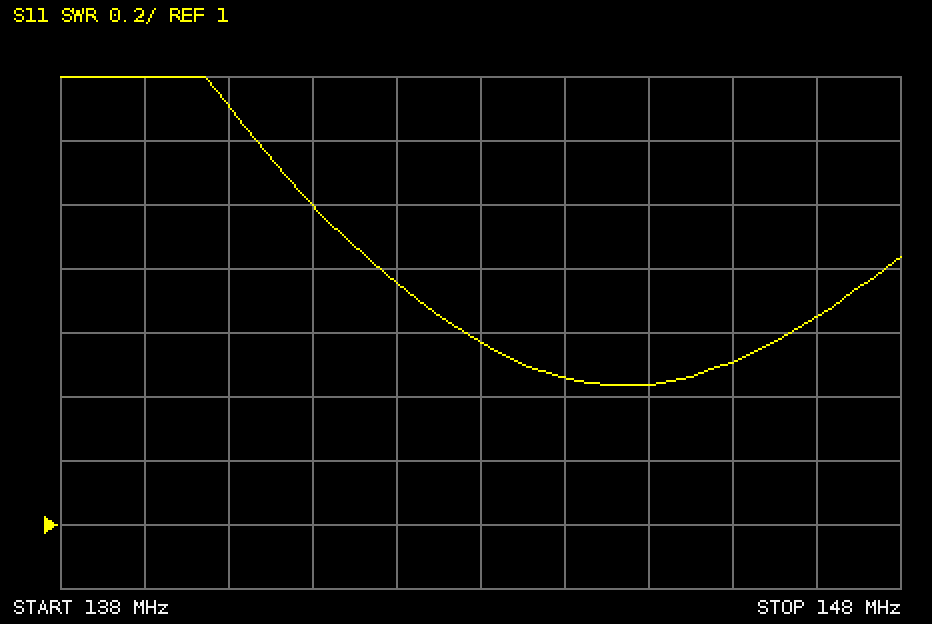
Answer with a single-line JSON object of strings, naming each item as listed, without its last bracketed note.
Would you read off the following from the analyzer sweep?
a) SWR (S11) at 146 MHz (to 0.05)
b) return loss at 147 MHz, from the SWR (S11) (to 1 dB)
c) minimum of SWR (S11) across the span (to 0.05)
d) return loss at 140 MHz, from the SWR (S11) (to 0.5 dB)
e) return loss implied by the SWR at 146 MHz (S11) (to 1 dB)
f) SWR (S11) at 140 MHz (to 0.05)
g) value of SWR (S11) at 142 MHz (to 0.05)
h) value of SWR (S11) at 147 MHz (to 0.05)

{"SWR (S11) at 146 MHz": "1.50", "return loss at 147 MHz, from the SWR (S11)": "12 dB", "minimum of SWR (S11) across the span": "1.45", "return loss at 140 MHz, from the SWR (S11)": "8.0 dB", "return loss implied by the SWR at 146 MHz (S11)": "14 dB", "SWR (S11) at 140 MHz": "2.30", "value of SWR (S11) at 142 MHz": "1.75", "value of SWR (S11) at 147 MHz": "1.65"}
